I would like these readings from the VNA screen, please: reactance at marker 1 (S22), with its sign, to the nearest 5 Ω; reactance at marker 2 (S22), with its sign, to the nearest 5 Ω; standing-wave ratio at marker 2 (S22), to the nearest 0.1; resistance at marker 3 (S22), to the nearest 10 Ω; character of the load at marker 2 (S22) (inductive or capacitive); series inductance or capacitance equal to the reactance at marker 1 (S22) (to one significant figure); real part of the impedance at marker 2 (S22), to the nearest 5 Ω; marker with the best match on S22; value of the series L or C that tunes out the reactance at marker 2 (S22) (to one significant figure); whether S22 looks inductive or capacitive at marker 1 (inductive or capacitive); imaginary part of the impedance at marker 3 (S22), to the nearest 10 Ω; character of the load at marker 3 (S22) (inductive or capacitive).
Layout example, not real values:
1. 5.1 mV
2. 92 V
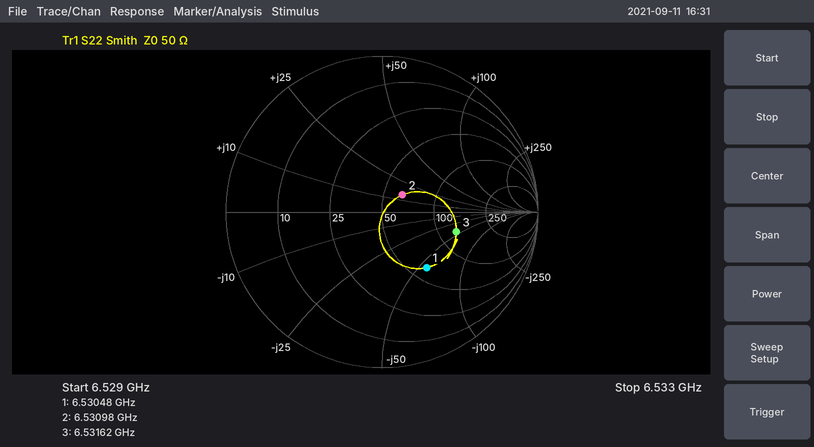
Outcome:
1. -55 Ω
2. +15 Ω
3. 1.4
4. 130 Ω
5. inductive
6. 400 fF
7. 65 Ω
8. marker 2
9. 2 pF
10. capacitive
11. -40 Ω
12. capacitive
